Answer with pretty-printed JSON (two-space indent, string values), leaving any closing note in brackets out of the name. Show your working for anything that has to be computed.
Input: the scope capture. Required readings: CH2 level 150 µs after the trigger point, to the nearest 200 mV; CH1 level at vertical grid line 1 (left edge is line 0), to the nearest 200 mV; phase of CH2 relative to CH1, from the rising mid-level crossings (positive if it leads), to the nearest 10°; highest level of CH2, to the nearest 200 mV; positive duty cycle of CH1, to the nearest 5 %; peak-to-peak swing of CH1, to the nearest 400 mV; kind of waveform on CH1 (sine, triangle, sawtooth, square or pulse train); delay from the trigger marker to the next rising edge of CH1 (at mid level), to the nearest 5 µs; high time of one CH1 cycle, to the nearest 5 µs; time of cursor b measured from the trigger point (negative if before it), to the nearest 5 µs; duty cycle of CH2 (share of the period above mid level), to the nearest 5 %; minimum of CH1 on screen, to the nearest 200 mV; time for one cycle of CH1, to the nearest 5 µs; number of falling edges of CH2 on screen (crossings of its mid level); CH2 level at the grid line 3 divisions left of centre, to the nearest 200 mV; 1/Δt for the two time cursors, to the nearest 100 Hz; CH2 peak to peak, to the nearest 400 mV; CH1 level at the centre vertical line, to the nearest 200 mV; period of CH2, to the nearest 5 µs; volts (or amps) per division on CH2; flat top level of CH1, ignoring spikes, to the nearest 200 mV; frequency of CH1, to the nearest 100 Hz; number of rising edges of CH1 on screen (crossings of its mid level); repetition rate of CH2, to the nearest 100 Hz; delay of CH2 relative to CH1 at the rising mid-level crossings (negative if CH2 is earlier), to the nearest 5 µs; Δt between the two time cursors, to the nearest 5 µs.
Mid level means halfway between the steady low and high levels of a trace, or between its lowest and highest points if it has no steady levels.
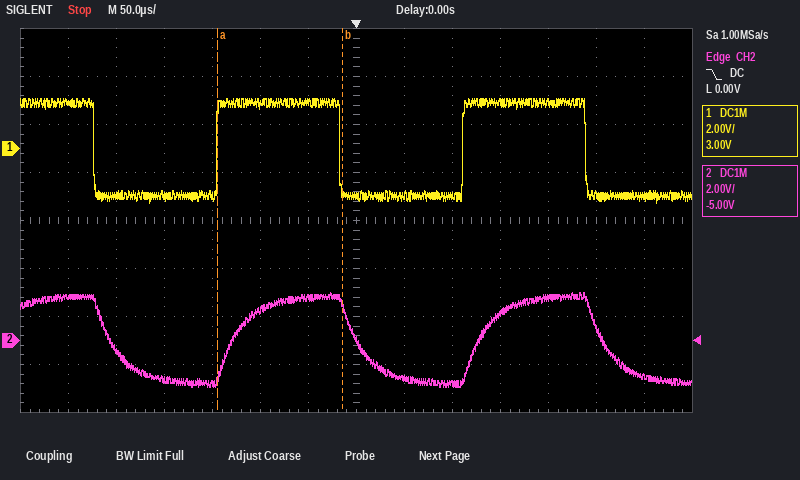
{
  "CH2 level 150 µs after the trigger point, to the nearest 200 mV": "1.2 V",
  "CH1 level at vertical grid line 1 (left edge is line 0), to the nearest 200 mV": "2.0 V",
  "phase of CH2 relative to CH1, from the rising mid-level crossings (positive if it leads), to the nearest 10°": "−360° × (+15 µs) / 255 µs ≈ -21.2°, so -20° to the nearest 10°",
  "highest level of CH2, to the nearest 200 mV": "2.0 V",
  "positive duty cycle of CH1, to the nearest 5 %": "130 µs / 255 µs ≈ 51.0 %, so 50 % to the nearest 5 %",
  "peak-to-peak swing of CH1, to the nearest 400 mV": "4.4 V",
  "kind of waveform on CH1": "square",
  "delay from the trigger marker to the next rising edge of CH1 (at mid level), to the nearest 5 µs": "110 µs",
  "high time of one CH1 cycle, to the nearest 5 µs": "130 µs",
  "time of cursor b measured from the trigger point (negative if before it), to the nearest 5 µs": "-15 µs",
  "duty cycle of CH2 (share of the period above mid level), to the nearest 5 %": "50 %",
  "minimum of CH1 on screen, to the nearest 200 mV": "-2.2 V",
  "time for one cycle of CH1, to the nearest 5 µs": "255 µs",
  "number of falling edges of CH2 on screen": "3",
  "CH2 level at the grid line 3 divisions left of centre, to the nearest 200 mV": "-1.8 V",
  "1/Δt for the two time cursors, to the nearest 100 Hz": "1 / 130 µs ≈ 7.7 kHz",
  "CH2 peak to peak, to the nearest 400 mV": "4.0 V",
  "CH1 level at the centre vertical line, to the nearest 200 mV": "-2.0 V",
  "period of CH2, to the nearest 5 µs": "255 µs",
  "volts (or amps) per division on CH2": "2 V",
  "flat top level of CH1, ignoring spikes, to the nearest 200 mV": "2.0 V",
  "frequency of CH1, to the nearest 100 Hz": "1 / 255 µs ≈ 3.9 kHz",
  "number of rising edges of CH1 on screen": "2",
  "repetition rate of CH2, to the nearest 100 Hz": "1 / 255 µs ≈ 3.9 kHz",
  "delay of CH2 relative to CH1 at the rising mid-level crossings (negative if CH2 is earlier), to the nearest 5 µs": "+15 µs",
  "Δt between the two time cursors, to the nearest 5 µs": "130 µs"
}
